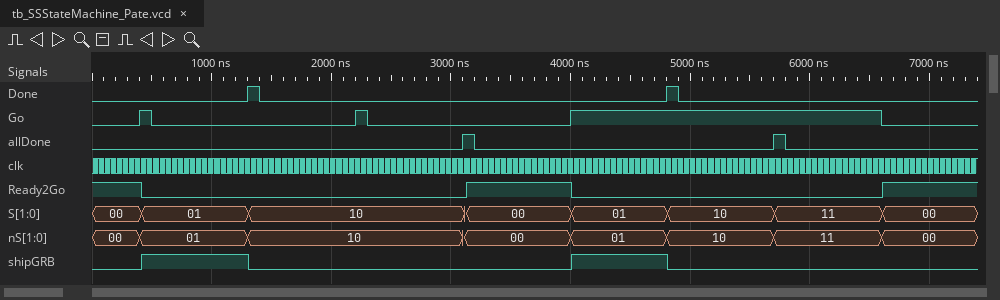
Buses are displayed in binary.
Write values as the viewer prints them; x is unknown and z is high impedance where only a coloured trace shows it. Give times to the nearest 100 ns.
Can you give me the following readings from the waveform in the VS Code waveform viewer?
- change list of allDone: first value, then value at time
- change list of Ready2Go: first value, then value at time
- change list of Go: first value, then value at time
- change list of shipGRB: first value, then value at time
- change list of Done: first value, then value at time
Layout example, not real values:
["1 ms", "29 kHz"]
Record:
["0, 1 at 3100 ns, 0 at 3200 ns, 1 at 5700 ns, 0 at 5800 ns", "1, 0 at 400 ns, 1 at 3100 ns, 0 at 4000 ns, 1 at 6600 ns", "0, 1 at 400 ns, 0 at 500 ns, 1 at 2200 ns, 0 at 2300 ns, 1 at 4000 ns, 0 at 6600 ns", "0, 1 at 400 ns, 0 at 1300 ns, 1 at 4000 ns, 0 at 4800 ns", "0, 1 at 1300 ns, 0 at 1400 ns, 1 at 4800 ns, 0 at 4900 ns"]
